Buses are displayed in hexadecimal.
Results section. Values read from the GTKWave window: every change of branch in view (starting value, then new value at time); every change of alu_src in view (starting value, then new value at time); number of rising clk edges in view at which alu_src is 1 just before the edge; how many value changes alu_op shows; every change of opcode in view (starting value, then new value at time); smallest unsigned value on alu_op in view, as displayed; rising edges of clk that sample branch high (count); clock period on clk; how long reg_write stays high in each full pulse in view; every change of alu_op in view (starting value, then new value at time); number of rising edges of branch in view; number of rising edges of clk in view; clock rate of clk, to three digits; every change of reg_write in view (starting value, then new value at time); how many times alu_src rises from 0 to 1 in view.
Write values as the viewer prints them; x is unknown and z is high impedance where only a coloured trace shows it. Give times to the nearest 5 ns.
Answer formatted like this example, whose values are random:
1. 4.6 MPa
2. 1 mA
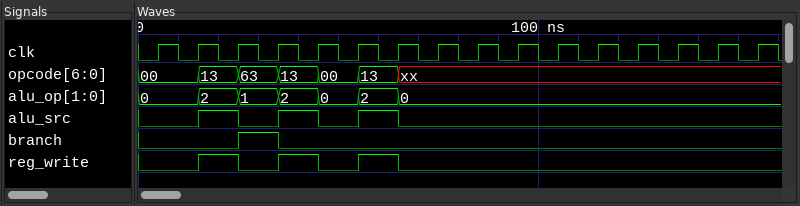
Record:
1. 0, 1 at 25 ns, 0 at 35 ns
2. 0, 1 at 15 ns, 0 at 25 ns, 1 at 35 ns, 0 at 45 ns, 1 at 55 ns, 0 at 65 ns
3. 3
4. 6
5. 00, 13 at 15 ns, 63 at 25 ns, 13 at 35 ns, 00 at 45 ns, 13 at 55 ns, xx at 65 ns
6. 0
7. 1
8. 10 ns
9. 10 ns, 10 ns, 10 ns
10. 0, 2 at 15 ns, 1 at 25 ns, 2 at 35 ns, 0 at 45 ns, 2 at 55 ns, 0 at 65 ns
11. 1
12. 16
13. 100 MHz
14. 0, 1 at 15 ns, 0 at 25 ns, 1 at 35 ns, 0 at 45 ns, 1 at 55 ns, 0 at 65 ns
15. 3
